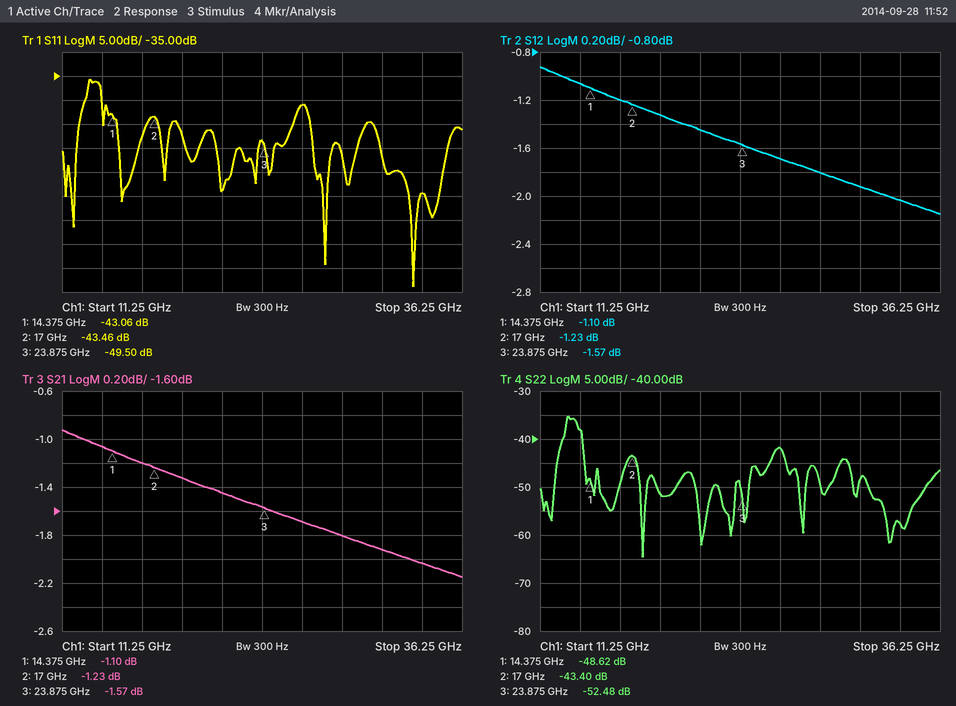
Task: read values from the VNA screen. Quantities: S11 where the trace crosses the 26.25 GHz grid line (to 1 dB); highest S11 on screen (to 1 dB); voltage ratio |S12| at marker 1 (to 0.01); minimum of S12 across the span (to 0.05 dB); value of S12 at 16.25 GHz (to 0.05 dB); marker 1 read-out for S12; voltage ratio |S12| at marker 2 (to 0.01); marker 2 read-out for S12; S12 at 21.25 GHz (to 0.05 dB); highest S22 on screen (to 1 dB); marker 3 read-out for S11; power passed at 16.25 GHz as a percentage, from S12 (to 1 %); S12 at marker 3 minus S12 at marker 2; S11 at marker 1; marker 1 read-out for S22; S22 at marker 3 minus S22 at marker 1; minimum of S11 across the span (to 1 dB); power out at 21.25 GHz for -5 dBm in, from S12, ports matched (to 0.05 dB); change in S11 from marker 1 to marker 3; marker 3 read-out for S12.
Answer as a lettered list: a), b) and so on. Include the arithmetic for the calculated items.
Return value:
a) -41 dB
b) -36 dB
c) 10^(-1.1/20) ≈ 0.88
d) -2.15 dB
e) -1.20 dB
f) -1.10 dB
g) 10^(-1.23/20) ≈ 0.87
h) -1.23 dB
i) -1.45 dB
j) -35 dB
k) -49.50 dB
l) 10^(-1.2/10) ≈ 76 %
m) -1.57 − (-1.23) = -0.34 dB
n) -43.06 dB
o) -48.62 dB
p) -52.48 − (-48.62) = -3.86 dB
q) -79 dB
r) -5 dBm + (-1.45 dB) = -6.45 dBm
s) -49.5 − (-43.06) = -6.44 dB
t) -1.57 dB
